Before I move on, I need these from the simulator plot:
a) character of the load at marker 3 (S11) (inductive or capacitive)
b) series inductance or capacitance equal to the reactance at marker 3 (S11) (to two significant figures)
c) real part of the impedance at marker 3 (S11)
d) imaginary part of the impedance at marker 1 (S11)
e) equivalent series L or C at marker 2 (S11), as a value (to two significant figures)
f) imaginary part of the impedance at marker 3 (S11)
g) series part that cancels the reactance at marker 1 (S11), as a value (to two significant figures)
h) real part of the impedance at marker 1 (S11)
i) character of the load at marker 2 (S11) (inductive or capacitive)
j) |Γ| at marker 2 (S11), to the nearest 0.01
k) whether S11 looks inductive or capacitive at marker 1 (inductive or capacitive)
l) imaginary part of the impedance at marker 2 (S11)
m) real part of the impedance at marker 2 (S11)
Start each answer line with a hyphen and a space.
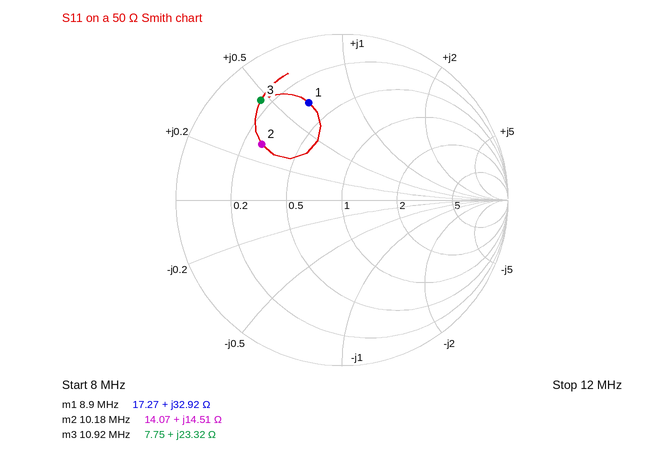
- inductive
- 340 nH
- 7.75 Ω
- +32.92 Ω
- 230 nH
- +23.32 Ω
- 540 pF
- 17.27 Ω
- inductive
- 0.59
- inductive
- +14.51 Ω
- 14.07 Ω
